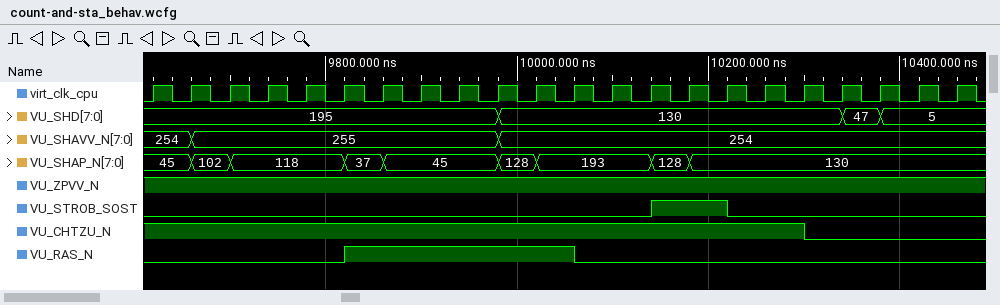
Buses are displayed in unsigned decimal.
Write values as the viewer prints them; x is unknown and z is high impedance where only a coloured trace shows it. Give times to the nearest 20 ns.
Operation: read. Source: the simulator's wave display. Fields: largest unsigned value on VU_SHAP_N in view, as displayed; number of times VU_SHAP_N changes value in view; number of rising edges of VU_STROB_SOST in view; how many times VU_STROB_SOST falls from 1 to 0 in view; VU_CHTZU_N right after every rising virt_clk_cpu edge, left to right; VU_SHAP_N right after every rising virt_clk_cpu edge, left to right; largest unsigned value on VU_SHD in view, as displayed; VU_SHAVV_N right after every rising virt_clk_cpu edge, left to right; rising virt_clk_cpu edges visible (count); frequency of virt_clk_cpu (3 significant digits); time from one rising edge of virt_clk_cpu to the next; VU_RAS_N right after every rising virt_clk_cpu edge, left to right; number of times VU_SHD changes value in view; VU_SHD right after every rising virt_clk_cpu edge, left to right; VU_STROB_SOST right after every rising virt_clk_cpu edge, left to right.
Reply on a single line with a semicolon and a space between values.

193; 8; 1; 1; 1 1 1 1 1 1 1 1 1 1 1 1 1 1 1 1 1 0 0 0 0 0; 45, 102, 118, 118, 118, 37, 45, 45, 45, 128, 193, 193, 193, 128, 130, 130, 130, 130, 130, 130, 130, 130; 195; 254, 255, 255, 255, 255, 255, 255, 255, 255, 254, 254, 254, 254, 254, 254, 254, 254, 254, 254, 254, 254, 254; 22; 25.0 MHz; 40 ns; 0 0 0 0 0 1 1 1 1 1 1 0 0 0 0 0 0 0 0 0 0 0; 3; 195, 195, 195, 195, 195, 195, 195, 195, 195, 130, 130, 130, 130, 130, 130, 130, 130, 130, 47, 5, 5, 5; 0 0 0 0 0 0 0 0 0 0 0 0 0 1 1 0 0 0 0 0 0 0
